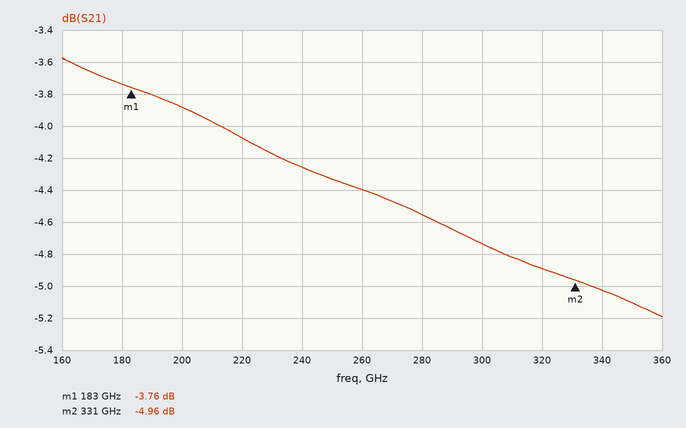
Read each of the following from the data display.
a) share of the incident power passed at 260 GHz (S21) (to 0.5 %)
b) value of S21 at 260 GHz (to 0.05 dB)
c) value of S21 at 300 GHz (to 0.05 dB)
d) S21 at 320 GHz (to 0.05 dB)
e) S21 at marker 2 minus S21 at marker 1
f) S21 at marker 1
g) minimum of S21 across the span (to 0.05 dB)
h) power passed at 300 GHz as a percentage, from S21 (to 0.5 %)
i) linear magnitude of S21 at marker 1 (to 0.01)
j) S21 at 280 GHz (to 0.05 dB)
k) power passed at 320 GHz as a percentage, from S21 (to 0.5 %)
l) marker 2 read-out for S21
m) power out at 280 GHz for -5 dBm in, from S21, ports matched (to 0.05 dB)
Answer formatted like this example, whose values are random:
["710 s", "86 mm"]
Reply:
["36.5 %", "-4.40 dB", "-4.75 dB", "-4.90 dB", "-1.20 dB", "-3.76 dB", "-5.20 dB", "33.5 %", "0.65", "-4.55 dB", "32.5 %", "-4.96 dB", "-9.55 dBm"]
